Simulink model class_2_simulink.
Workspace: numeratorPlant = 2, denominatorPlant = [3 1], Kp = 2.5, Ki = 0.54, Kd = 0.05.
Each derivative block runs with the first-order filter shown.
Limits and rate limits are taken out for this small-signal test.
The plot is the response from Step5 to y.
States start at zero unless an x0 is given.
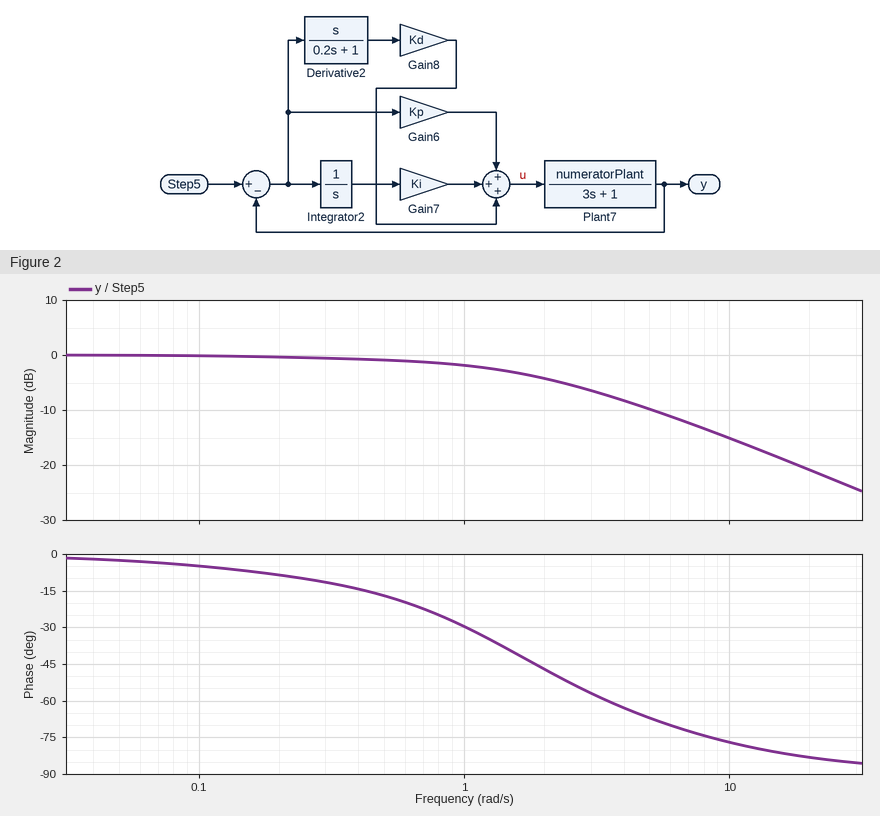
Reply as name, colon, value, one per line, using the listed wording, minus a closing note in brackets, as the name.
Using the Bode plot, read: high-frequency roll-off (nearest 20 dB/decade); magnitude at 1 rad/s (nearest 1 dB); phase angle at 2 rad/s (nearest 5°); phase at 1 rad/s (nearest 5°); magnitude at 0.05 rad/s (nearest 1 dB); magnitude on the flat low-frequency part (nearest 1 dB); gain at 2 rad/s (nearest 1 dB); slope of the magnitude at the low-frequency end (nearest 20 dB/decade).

high-frequency roll-off: -20 dB/decade
magnitude at 1 rad/s: -2 dB
phase angle at 2 rad/s: -45°
phase at 1 rad/s: -30°
magnitude at 0.05 rad/s: 0 dB
magnitude on the flat low-frequency part: 0 dB
gain at 2 rad/s: -4 dB
slope of the magnitude at the low-frequency end: 0 dB/decade
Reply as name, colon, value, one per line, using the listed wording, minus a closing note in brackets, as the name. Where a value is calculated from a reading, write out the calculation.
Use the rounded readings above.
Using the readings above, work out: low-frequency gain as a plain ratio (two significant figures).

low-frequency gain as a plain ratio: 10^(0 / 20) = 1.0
